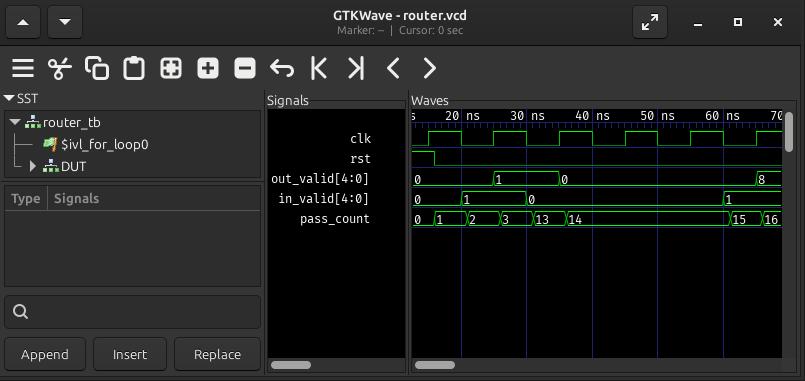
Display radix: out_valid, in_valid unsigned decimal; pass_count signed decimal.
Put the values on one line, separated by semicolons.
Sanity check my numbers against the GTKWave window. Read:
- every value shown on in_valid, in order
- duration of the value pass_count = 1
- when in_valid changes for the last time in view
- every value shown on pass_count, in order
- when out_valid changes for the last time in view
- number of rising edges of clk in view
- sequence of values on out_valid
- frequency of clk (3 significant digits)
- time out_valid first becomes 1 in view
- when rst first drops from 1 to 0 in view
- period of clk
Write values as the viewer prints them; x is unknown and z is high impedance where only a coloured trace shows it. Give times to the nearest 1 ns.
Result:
0, 1, 0, 1; 5 ns; 60 ns; 0, 1, 2, 3, 13, 14, 15, 16; 65 ns; 6; 0, 1, 0, 8; 100 MHz; 25 ns; 16 ns; 10 ns
